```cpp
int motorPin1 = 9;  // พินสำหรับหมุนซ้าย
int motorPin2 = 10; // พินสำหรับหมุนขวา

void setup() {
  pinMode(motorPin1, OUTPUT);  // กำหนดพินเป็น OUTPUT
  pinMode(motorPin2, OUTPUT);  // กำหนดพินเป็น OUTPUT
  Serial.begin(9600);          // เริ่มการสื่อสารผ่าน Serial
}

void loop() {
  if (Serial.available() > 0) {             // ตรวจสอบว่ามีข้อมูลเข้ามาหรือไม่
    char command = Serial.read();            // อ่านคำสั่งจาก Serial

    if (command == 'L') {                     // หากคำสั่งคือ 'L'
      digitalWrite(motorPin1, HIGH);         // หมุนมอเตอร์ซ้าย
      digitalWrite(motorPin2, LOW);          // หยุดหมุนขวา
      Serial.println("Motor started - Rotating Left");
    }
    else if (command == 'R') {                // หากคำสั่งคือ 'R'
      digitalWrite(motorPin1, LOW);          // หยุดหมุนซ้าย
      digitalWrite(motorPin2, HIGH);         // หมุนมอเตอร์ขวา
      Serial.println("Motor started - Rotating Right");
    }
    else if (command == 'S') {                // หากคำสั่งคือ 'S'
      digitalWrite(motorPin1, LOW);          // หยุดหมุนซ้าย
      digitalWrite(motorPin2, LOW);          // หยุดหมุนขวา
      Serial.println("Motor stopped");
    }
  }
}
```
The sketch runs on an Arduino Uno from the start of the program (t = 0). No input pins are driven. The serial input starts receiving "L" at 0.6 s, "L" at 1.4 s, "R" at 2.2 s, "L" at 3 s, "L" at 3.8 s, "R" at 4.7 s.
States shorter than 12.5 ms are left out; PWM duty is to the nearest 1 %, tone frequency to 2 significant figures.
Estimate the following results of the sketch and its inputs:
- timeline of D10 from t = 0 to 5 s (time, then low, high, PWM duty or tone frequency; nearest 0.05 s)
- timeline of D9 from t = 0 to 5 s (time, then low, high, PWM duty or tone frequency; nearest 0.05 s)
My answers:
0 s low; 2.2 s high; 3 s low; 4.7 s high
0 s low; 0.6 s high; 2.2 s low; 3 s high; 4.7 s low
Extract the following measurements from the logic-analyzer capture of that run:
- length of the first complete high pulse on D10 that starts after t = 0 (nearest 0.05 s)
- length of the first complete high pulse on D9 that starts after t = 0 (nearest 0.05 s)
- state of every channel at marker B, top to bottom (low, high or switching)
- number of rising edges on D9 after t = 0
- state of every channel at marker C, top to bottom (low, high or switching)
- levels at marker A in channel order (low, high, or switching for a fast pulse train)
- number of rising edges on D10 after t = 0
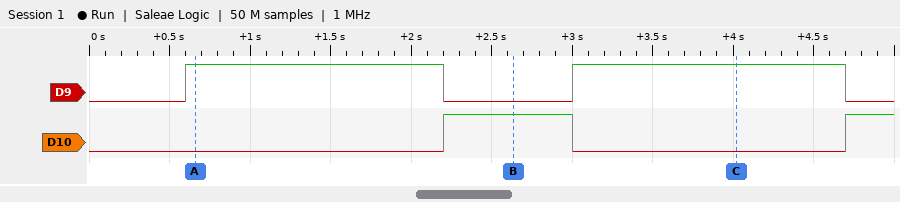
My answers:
0.80 s
1.60 s
D9 low, D10 high
2
D9 high, D10 low
D9 high, D10 low
2
